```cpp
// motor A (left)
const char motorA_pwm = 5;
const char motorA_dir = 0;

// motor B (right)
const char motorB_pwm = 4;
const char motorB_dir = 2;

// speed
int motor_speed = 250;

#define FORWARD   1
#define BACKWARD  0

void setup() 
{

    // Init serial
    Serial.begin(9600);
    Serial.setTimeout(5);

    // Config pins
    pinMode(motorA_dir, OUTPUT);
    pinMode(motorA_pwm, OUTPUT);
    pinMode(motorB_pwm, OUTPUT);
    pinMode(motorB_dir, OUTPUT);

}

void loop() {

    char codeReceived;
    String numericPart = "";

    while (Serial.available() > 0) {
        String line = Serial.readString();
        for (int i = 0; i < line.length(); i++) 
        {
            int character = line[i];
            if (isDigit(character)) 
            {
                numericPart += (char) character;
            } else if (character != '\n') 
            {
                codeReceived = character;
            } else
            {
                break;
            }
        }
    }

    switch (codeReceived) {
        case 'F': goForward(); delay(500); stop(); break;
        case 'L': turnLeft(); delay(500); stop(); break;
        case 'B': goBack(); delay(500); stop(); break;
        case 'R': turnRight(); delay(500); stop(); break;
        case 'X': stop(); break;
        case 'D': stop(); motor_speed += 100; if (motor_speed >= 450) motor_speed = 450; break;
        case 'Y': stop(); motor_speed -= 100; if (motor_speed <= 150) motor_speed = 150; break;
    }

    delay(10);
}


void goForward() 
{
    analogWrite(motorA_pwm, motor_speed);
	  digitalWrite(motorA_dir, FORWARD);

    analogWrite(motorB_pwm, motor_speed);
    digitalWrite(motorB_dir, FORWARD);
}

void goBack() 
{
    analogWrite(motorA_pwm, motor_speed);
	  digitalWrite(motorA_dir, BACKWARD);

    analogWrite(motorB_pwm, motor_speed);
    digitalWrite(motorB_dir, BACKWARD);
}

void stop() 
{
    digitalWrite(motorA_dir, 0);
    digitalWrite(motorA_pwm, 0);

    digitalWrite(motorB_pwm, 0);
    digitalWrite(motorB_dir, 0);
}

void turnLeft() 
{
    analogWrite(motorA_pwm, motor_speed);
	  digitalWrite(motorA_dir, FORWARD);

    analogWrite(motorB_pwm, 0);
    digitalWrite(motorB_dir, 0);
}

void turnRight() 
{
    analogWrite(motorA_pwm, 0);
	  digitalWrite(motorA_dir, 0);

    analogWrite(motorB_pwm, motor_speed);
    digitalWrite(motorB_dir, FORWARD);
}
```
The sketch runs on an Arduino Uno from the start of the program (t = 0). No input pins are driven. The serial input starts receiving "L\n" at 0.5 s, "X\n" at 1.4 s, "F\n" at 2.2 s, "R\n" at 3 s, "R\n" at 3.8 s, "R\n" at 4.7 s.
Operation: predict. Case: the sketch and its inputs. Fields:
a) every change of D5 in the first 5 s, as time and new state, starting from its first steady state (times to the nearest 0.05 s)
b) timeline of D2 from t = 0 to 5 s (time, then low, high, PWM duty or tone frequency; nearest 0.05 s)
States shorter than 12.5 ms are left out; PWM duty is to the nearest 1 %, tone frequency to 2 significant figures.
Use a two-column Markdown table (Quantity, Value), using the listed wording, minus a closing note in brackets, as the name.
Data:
| Quantity | Value |
|---|---|
| every change of D5 in the first 5 s, as time and new state, starting from its first steady state | 0 s low; 0.5 s PWM 98 %; 1 s low; 2.2 s PWM 98 %; 2.7 s low |
| timeline of D2 from t = 0 to 5 s | 0 s low; 2.2 s high; 2.7 s low; 3 s high; 3.5 s low; 3.8 s high; 4.3 s low; 4.7 s high |
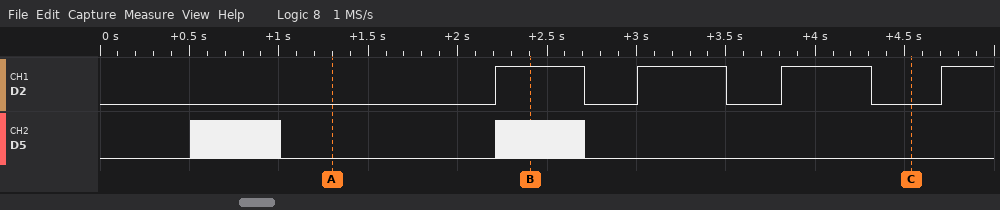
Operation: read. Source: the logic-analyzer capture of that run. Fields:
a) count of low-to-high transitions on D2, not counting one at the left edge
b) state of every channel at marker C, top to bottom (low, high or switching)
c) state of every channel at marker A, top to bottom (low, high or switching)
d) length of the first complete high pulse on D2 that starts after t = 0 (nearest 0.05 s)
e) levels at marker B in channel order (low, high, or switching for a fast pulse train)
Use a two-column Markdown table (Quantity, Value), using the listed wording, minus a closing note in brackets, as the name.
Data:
| Quantity | Value |
|---|---|
| count of low-to-high transitions on D2, not counting one at the left edge | 4 |
| state of every channel at marker C, top to bottom | D2 low, D5 low |
| state of every channel at marker A, top to bottom | D2 low, D5 low |
| length of the first complete high pulse on D2 that starts after t = 0 | 0.50 s |
| levels at marker B in channel order | D2 high, D5 switching |
